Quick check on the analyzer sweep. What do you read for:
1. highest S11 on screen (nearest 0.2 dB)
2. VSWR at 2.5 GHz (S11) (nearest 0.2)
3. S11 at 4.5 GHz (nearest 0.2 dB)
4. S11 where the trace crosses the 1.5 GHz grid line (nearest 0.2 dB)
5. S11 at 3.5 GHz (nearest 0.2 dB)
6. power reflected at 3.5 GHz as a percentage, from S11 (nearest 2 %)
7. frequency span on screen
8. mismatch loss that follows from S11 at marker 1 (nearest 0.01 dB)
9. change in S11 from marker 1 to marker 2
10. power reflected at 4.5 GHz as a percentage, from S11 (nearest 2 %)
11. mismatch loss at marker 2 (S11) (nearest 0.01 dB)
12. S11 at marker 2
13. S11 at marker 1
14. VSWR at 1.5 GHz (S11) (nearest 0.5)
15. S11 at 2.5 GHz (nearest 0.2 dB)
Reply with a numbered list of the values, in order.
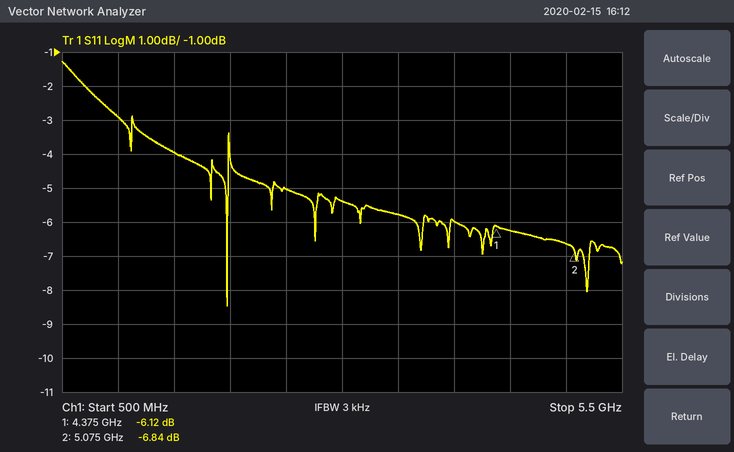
1. -1.2 dB
2. 3.6
3. -6.2 dB
4. -4.0 dB
5. -5.8 dB
6. 26 %
7. 5 GHz
8. 1.22 dB
9. -0.72 dB
10. 24 %
11. 1.01 dB
12. -6.84 dB
13. -6.12 dB
14. 4.5
15. -5.0 dB
